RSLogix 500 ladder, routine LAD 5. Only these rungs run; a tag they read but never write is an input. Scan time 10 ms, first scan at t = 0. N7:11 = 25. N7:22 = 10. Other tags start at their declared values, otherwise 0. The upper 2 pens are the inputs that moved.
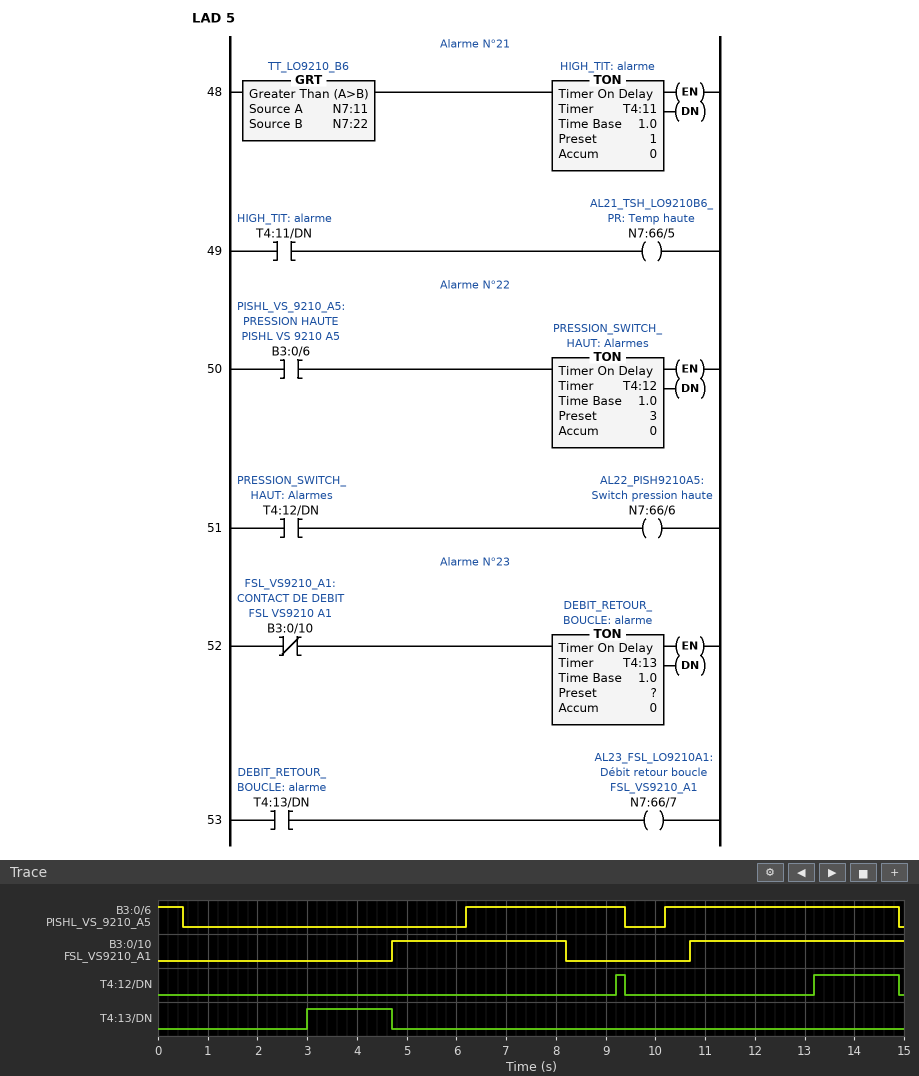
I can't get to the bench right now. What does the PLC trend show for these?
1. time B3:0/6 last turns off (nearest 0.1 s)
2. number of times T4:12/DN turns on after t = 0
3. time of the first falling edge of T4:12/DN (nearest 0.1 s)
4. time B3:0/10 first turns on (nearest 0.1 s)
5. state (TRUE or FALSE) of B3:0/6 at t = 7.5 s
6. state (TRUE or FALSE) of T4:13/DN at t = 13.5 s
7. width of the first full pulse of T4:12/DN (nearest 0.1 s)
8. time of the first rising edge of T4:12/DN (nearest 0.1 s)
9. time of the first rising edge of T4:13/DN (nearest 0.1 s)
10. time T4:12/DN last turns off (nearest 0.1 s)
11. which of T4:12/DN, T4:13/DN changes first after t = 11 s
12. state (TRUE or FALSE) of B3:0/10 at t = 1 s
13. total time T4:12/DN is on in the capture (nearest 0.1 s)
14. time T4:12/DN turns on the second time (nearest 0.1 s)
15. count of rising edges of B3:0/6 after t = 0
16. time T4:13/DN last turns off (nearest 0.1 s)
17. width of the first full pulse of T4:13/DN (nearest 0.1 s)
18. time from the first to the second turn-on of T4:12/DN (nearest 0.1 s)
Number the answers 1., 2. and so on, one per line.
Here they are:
1. 14.9 s
2. 2
3. 9.4 s
4. 4.7 s
5. TRUE
6. FALSE
7. 0.2 s
8. 9.2 s
9. 3.0 s
10. 14.9 s
11. T4:12/DN
12. FALSE
13. 1.9 s
14. 13.2 s
15. 2
16. 4.7 s
17. 1.7 s
18. 4.0 s
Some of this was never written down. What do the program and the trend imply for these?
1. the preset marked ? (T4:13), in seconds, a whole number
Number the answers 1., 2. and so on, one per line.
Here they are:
1. 3 s
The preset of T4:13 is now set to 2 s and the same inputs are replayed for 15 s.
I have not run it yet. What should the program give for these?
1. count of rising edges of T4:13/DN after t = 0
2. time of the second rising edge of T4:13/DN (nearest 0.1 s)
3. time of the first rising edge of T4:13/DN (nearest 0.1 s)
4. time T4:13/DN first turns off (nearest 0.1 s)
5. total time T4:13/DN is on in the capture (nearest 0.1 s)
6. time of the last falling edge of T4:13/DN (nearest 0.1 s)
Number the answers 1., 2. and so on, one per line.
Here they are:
1. 2
2. 10.2 s
3. 2.0 s
4. 4.7 s
5. 3.2 s
6. 10.7 s
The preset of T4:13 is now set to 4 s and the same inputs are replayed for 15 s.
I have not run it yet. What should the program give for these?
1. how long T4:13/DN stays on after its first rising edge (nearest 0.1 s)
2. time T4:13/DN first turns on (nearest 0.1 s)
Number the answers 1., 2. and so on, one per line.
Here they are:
1. 0.7 s
2. 4.0 s
